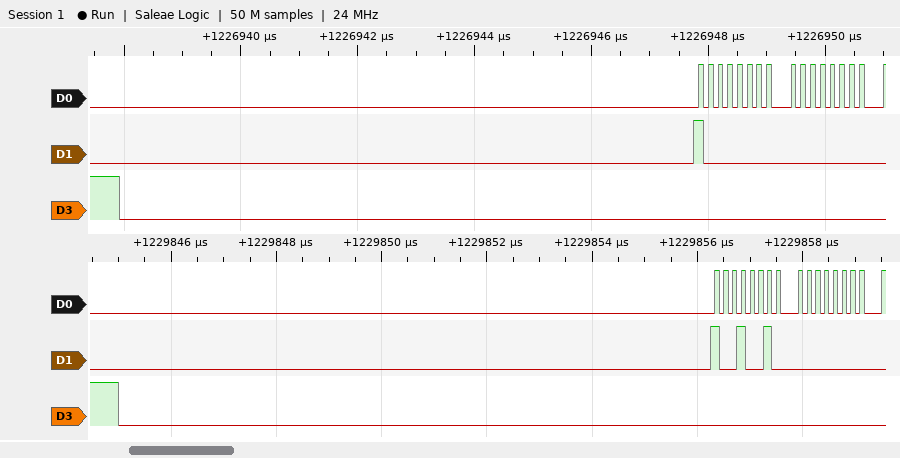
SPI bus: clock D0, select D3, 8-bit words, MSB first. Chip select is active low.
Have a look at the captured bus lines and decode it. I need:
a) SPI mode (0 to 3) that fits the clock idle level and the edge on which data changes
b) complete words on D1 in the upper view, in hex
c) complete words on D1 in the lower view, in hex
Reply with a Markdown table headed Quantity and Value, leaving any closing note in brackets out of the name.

| Quantity | Value |
|---|---|
| SPI mode (0 to 3) that fits the clock idle level and the edge on which data changes | 0 |
| complete words on D1 in the upper view, in hex | 80, 00 |
| complete words on D1 in the lower view, in hex | 92, 00 |
